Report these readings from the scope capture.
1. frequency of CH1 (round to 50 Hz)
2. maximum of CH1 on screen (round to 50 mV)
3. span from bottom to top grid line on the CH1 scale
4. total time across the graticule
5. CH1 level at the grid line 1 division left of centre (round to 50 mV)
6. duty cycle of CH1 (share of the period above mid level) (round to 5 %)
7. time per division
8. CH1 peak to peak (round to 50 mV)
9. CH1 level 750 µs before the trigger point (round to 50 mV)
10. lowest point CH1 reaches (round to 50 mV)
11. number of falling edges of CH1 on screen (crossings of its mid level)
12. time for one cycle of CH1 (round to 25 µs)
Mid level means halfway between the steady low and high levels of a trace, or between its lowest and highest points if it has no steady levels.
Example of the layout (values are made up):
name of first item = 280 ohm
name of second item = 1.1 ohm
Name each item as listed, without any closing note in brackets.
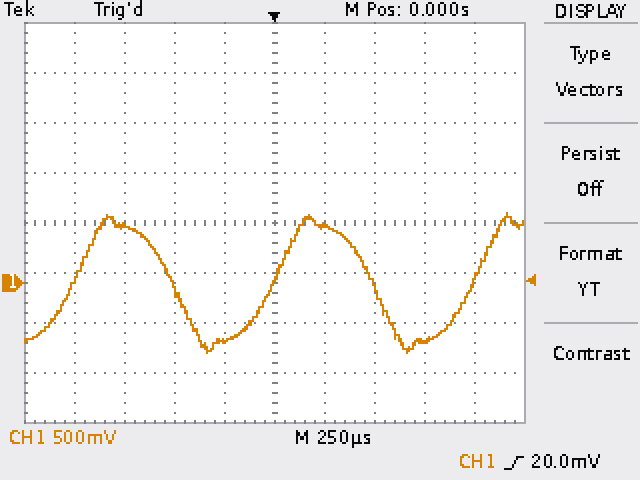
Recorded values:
frequency of CH1 = 1.00 kHz
maximum of CH1 on screen = 700 mV
span from bottom to top grid line on the CH1 scale = 4 V
total time across the graticule = 2.5 ms
CH1 level at the grid line 1 division left of centre = -600 mV
duty cycle of CH1 (share of the period above mid level) = 50 %
time per division = 250 µs
CH1 peak to peak = 1.40 V
CH1 level 750 µs before the trigger point = 550 mV
lowest point CH1 reaches = -700 mV
number of falling edges of CH1 on screen = 2
time for one cycle of CH1 = 1.000 ms
